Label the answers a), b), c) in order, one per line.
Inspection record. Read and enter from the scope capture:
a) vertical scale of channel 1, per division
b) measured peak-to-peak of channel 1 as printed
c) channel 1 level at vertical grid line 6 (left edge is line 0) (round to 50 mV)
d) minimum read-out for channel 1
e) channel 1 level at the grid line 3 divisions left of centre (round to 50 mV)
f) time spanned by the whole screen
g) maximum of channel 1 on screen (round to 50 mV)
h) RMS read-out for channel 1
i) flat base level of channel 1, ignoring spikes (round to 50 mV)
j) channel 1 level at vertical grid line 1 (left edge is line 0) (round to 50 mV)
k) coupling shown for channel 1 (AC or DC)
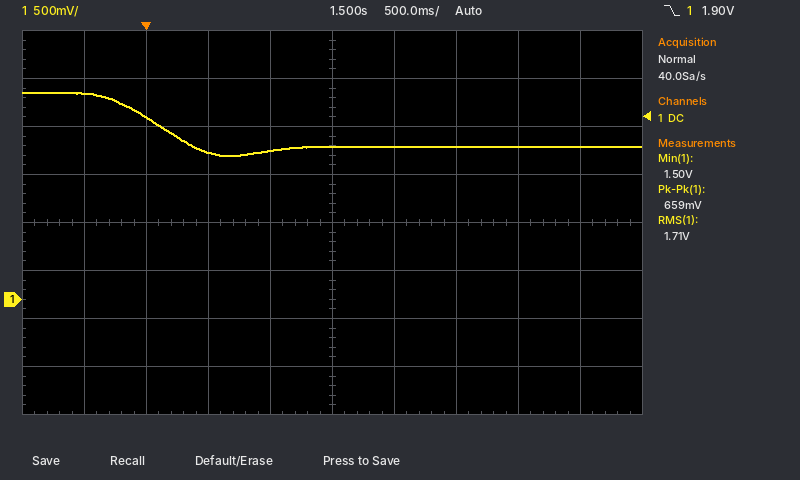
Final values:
a) 500 mV
b) 659 mV
c) 1.60 V
d) 1.50 V
e) 1.90 V
f) 5 s
g) 2.15 V
h) 1.71 V
i) 1.60 V
j) 2.15 V
k) DC
